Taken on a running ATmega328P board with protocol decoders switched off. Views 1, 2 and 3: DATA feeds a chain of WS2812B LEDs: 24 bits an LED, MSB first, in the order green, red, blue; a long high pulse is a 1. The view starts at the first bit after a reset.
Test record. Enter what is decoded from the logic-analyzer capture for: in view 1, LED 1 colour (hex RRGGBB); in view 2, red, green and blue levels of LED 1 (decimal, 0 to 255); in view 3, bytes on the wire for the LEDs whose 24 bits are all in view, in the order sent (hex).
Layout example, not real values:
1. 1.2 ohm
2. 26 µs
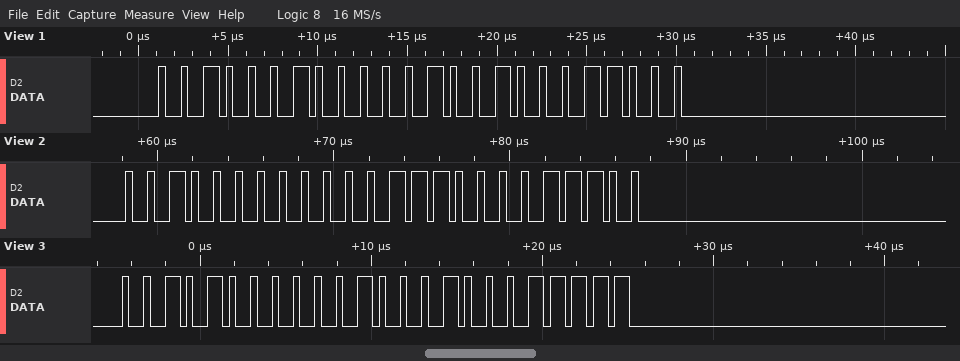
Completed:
1. #092218
2. 14, 32, 28
3. 28 11 1F
